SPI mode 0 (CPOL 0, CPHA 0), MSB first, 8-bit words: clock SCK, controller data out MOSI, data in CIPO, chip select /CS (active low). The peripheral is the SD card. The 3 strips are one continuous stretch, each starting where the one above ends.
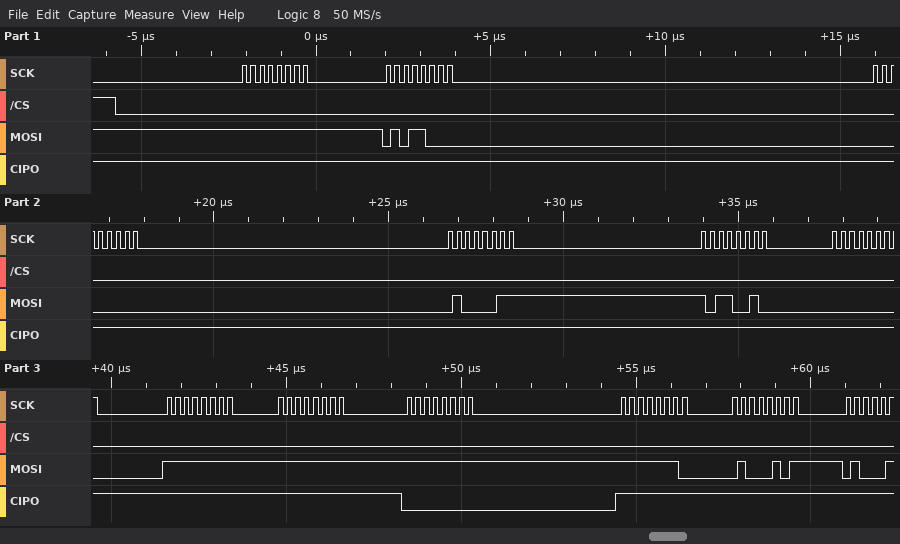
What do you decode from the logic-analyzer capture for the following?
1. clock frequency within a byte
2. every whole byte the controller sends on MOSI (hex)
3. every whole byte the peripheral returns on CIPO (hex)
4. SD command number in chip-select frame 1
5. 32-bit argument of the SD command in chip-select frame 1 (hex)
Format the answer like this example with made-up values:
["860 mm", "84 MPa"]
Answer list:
["4 MHz", "0xFF 0x58 0x00 0x43 0xB2 0x00 0xFF 0xFF 0xFF 0xFE 0x45", "0xFF 0xFF 0xFF 0xFF 0xFF 0xFF 0xFF 0xFF 0x00 0xFF 0xFF", "CMD24", "0x0043B200"]
